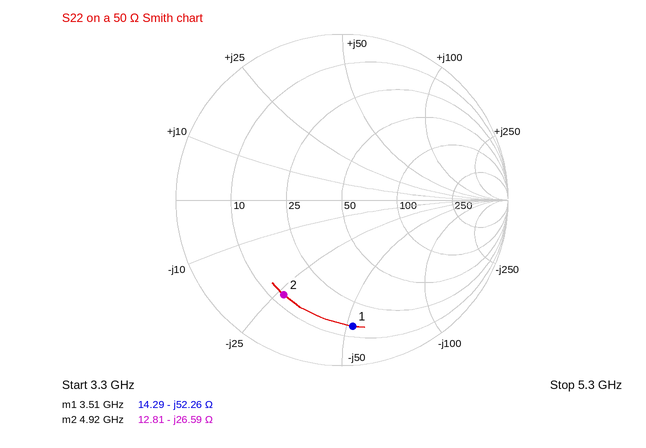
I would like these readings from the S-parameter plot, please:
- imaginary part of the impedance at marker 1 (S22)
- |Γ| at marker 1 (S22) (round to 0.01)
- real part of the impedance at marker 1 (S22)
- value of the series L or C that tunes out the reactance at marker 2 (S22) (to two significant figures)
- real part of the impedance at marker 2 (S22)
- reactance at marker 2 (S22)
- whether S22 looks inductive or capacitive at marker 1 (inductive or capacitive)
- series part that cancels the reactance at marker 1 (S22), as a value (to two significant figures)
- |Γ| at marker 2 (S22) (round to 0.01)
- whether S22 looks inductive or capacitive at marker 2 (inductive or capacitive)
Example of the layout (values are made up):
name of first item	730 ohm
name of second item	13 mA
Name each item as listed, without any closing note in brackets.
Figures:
imaginary part of the impedance at marker 1	-52.26 Ω
|Γ| at marker 1 (S22)	0.76
real part of the impedance at marker 1	14.29 Ω
value of the series L or C that tunes out the reactance at marker 2 (S22)	860 pH
real part of the impedance at marker 2	12.81 Ω
reactance at marker 2	-26.59 Ω
whether S22 looks inductive or capacitive at marker 1	capacitive
series part that cancels the reactance at marker 1 (S22), as a value	2.4 nH
|Γ| at marker 2 (S22)	0.67
whether S22 looks inductive or capacitive at marker 2	capacitive
